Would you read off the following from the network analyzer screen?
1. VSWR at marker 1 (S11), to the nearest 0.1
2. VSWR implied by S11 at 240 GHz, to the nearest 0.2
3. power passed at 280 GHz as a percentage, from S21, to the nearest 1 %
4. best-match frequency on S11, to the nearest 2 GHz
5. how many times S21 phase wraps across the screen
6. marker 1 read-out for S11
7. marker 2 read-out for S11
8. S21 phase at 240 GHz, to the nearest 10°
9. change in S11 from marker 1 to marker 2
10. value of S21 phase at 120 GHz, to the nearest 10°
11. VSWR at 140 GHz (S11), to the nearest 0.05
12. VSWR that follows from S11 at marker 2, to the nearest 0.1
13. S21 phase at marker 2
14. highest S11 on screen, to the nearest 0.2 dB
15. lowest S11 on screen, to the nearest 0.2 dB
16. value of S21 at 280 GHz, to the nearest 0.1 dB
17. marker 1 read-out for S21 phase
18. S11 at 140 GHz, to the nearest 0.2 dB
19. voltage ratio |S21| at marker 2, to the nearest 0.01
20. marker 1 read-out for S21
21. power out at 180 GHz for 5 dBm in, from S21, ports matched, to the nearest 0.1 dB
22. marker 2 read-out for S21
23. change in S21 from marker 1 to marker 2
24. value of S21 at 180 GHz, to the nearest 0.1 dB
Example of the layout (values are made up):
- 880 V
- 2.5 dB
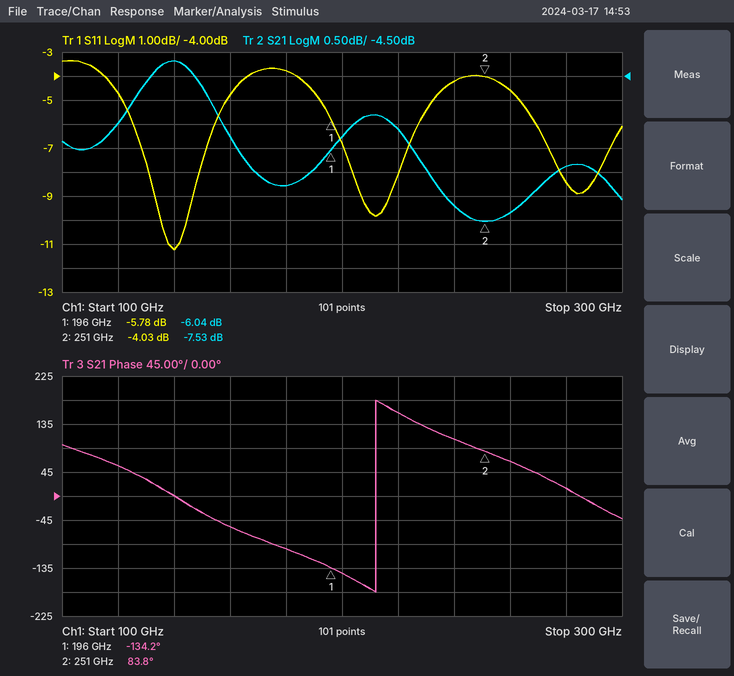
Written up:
- 3.1
- 4.2
- 23 %
- 140 GHz
- 1
- -5.78 dB
- -4.03 dB
- 110°
- 1.75 dB
- 60°
- 1.75
- 4.4
- 83.8°
- -3.4 dB
- -11.2 dB
- -6.4 dB
- -134.2°
- -11.2 dB
- 0.42
- -6.04 dB
- -1.8 dBm
- -7.53 dB
- -1.49 dB
- -6.8 dB
